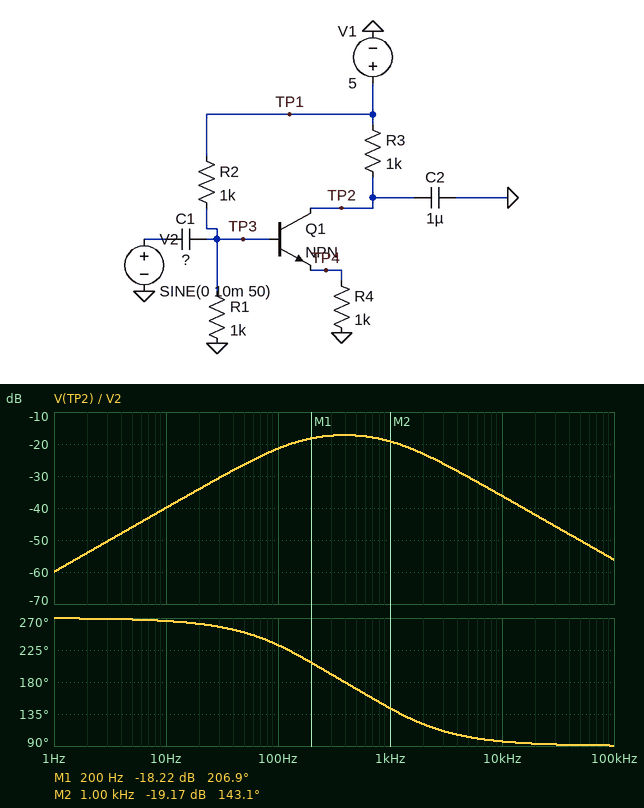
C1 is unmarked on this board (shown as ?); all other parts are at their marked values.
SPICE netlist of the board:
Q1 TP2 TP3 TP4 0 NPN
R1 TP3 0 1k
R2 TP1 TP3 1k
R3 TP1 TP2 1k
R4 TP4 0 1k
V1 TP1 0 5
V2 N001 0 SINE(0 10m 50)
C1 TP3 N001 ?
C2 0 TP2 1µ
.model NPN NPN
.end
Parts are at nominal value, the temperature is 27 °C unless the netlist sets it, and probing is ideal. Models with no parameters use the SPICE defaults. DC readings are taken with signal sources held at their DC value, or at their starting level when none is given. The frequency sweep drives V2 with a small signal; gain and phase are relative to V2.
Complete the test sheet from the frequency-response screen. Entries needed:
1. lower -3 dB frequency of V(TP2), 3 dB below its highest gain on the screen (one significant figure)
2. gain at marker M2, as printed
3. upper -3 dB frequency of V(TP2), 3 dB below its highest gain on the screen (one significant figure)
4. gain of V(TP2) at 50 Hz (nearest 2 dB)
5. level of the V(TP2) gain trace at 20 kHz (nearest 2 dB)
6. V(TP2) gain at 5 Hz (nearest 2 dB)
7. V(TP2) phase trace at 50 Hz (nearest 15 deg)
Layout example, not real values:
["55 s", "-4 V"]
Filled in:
["100 Hz", "-19.17 dB", "1 kHz", "-26 dB", "-42 dB", "-46 dB", "255 deg"]
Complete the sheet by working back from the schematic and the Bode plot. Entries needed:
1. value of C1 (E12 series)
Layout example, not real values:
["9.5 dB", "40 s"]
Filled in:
["330 nF"]
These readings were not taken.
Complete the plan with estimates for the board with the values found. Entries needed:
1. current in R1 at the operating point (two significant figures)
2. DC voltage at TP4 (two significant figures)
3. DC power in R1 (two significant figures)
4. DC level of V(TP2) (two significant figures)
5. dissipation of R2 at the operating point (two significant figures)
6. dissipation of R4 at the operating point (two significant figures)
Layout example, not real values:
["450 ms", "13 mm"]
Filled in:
["2.5 mA", "1.7 V", "6.2 mW", "3.3 V", "6.3 mW", "2.9 mW"]
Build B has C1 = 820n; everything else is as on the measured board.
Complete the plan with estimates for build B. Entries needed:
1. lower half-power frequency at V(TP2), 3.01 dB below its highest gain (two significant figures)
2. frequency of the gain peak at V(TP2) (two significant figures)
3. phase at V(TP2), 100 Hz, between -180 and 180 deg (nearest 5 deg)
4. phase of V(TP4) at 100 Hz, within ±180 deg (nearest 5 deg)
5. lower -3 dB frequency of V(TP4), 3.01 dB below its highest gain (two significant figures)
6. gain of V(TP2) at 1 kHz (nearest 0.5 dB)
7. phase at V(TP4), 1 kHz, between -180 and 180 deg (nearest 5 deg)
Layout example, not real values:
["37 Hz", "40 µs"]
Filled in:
["96 Hz", "250 Hz", "-135 deg", "75 deg", "390 Hz", "-17.0 dB", "20 deg"]
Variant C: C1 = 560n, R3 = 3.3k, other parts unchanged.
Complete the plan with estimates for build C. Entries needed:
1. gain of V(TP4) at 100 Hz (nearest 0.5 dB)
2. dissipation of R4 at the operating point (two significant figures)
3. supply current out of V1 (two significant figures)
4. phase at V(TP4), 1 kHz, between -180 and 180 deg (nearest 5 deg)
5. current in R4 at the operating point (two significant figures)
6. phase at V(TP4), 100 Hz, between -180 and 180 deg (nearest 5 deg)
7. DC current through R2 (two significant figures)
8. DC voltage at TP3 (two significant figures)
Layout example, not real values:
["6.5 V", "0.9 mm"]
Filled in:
["-20.0 dB", "2.2 mW", "3.8 mA", "25 deg", "1.5 mA", "75 deg", "2.7 mA", "2.3 V"]
